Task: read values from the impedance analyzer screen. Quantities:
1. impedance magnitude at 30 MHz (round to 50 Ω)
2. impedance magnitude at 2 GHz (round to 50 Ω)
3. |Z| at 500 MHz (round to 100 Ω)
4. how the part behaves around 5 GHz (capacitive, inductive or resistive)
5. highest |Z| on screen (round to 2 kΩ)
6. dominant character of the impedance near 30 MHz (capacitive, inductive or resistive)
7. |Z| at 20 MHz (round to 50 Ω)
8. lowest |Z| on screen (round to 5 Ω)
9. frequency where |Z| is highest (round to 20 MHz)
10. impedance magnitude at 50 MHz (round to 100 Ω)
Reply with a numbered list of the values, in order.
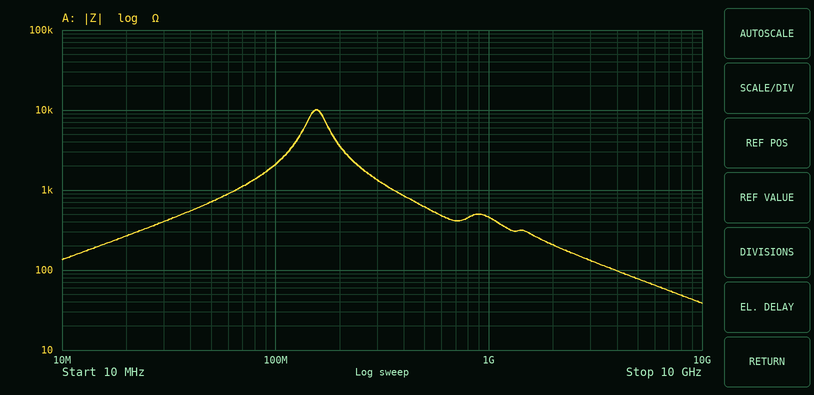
1. 400 Ω
2. 200 Ω
3. 600 Ω
4. capacitive
5. 10 kΩ
6. inductive
7. 250 Ω
8. 40 Ω
9. 160 MHz
10. 700 Ω
